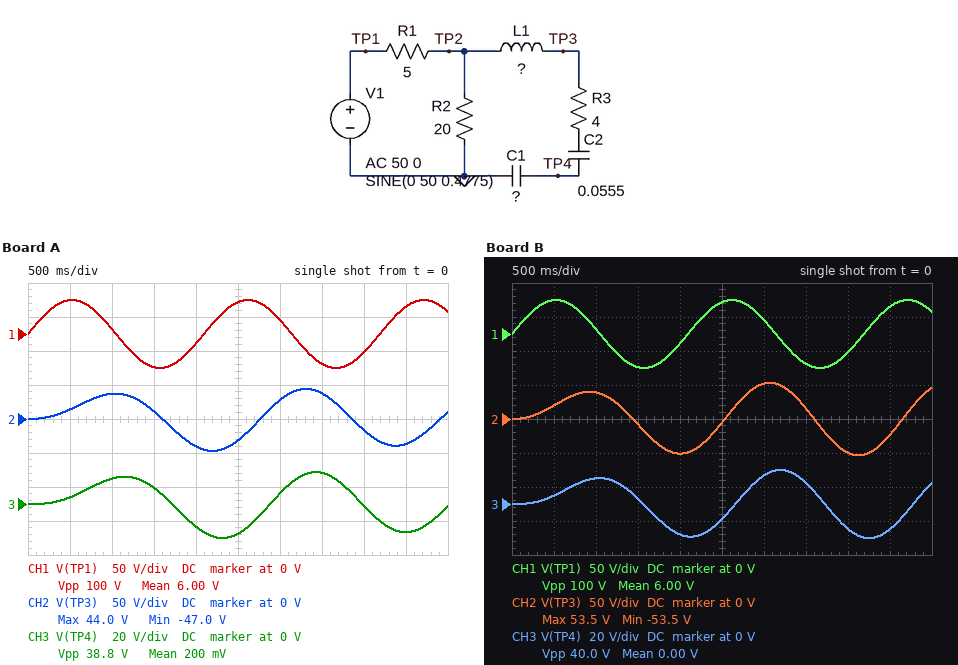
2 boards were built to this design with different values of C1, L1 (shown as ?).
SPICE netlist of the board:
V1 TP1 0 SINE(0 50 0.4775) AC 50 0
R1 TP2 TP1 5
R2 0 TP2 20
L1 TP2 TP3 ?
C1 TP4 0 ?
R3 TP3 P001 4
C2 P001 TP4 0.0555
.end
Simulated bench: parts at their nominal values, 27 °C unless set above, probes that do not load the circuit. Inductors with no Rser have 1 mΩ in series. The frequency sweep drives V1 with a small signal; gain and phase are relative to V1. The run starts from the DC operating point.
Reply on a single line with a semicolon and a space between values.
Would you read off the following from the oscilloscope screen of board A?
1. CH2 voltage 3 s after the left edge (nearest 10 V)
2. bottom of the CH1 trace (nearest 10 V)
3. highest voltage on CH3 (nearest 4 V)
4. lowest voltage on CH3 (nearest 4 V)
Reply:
30 V; -50 V; 20 V; -20 V
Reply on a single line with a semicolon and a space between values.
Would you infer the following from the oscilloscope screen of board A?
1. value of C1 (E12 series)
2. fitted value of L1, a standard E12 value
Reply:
68 mF; 6.8 H
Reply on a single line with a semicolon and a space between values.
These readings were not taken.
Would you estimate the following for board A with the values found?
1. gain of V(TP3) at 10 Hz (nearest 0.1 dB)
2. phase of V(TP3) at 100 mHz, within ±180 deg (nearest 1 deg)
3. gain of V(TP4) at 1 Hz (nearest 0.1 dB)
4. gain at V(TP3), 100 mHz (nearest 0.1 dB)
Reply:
-42.4 dB; -5 deg; -26.2 dB; -1.3 dB
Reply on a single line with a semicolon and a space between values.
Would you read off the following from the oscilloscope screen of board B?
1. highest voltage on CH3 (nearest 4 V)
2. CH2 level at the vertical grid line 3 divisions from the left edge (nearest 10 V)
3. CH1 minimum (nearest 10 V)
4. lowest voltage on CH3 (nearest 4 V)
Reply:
20 V; -10 V; -50 V; -20 V
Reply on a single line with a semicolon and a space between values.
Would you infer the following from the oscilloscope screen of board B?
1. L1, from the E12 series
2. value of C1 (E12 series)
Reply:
3.9 H; 82 mF
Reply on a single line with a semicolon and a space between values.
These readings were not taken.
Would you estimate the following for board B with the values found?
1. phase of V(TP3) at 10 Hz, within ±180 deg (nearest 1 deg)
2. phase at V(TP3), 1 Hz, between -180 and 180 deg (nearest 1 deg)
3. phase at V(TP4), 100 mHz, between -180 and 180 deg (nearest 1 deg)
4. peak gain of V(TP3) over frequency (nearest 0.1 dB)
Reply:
-95 deg; -118 deg; -10 deg; 1.8 dB
